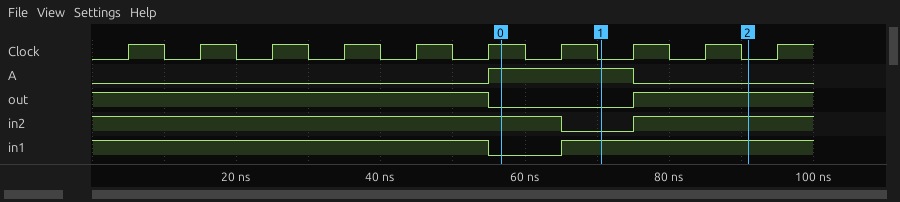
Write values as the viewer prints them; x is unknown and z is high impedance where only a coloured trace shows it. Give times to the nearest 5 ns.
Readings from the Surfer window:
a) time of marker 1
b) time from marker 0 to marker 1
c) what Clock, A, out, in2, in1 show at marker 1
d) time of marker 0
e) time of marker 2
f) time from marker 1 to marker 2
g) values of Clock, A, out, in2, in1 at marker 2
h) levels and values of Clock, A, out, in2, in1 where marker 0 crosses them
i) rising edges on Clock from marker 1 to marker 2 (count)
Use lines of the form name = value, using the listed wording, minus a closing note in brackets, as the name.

time of marker 1 = 70 ns
time from marker 0 to marker 1 = 15 ns
what Clock, A, out, in2, in1 show at marker 1 = Clock=0, A=1, out=0, in2=0, in1=1
time of marker 0 = 55 ns
time of marker 2 = 90 ns
time from marker 1 to marker 2 = 20 ns
values of Clock, A, out, in2, in1 at marker 2 = Clock=0, A=0, out=1, in2=1, in1=1
levels and values of Clock, A, out, in2, in1 where marker 0 crosses them = Clock=1, A=1, out=0, in2=1, in1=0
rising edges on Clock from marker 1 to marker 2 = 2
